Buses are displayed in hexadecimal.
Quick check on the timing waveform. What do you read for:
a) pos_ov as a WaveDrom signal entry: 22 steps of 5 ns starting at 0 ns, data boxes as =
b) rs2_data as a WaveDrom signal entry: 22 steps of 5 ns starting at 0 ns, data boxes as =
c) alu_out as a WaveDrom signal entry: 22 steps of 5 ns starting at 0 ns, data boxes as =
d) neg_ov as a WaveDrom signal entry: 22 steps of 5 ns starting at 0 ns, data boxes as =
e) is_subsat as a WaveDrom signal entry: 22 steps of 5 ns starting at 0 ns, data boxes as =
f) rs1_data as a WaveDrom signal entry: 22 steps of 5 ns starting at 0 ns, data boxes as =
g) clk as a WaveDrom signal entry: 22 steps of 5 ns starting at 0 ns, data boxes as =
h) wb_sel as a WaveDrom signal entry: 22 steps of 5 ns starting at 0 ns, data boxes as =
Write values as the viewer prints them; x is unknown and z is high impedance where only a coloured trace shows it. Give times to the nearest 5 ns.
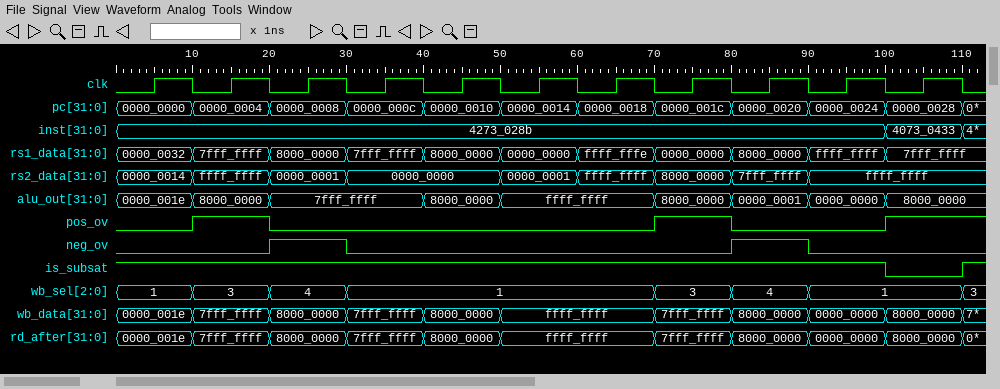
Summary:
{name: 'pos_ov', wave: '0.1.0.........1.0...1.'}
{name: 'rs2_data', wave: '=.=.=.=...=.=.=.=.=...', data: '0000_0014 ffff_ffff 0000_0001 0000_0000 0000_0001 ffff_ffff 8000_0000 7fff_ffff ffff_ffff'}
{name: 'alu_out', wave: '=.=.=...=.=...=.=.=.=.', data: '0000_001e 8000_0000 7fff_ffff 8000_0000 ffff_ffff 8000_0000 0000_0001 0000_0000 8000_0000'}
{name: 'neg_ov', wave: '0...1.0.........1.0...'}
{name: 'is_subsat', wave: '1...................0.'}
{name: 'rs1_data', wave: '=.=.=.=.=.=.=.=.=.=.=.', data: '0000_0032 7fff_ffff 8000_0000 7fff_ffff 8000_0000 0000_0000 ffff_fffe 0000_0000 8000_0000 ffff_ffff 7fff_ffff'}
{name: 'clk', wave: '0101010101010101010101'}
{name: 'wb_sel', wave: '=.=.=.=.......=.=.=...', data: '1 3 4 1 3 4 1'}
